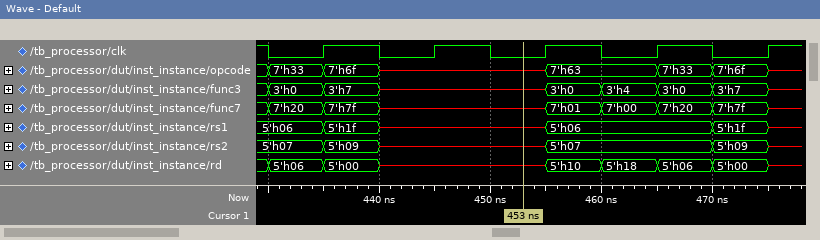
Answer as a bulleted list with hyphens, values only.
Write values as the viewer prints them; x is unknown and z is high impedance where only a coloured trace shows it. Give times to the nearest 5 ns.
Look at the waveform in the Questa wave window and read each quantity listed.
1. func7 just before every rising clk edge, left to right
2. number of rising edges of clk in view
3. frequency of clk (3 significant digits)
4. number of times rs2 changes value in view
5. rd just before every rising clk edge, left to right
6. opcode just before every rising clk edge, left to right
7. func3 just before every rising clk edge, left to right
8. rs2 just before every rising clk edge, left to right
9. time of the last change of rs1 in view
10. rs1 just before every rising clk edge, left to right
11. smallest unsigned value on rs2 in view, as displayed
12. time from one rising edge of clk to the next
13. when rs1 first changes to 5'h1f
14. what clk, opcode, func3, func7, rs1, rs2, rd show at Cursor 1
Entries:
- 7'h20, x, x, 7'h00, 7'h7f
- 5
- 100 MHz
- 5
- 5'h06, x, x, 5'h18, 5'h00
- 7'h33, x, x, 7'h63, 7'h6f
- 3'h0, x, x, 3'h4, 3'h7
- 5'h07, x, x, 5'h07, 5'h09
- 475 ns
- 5'h06, x, x, 5'h06, 5'h1f
- 5'h07
- 10 ns
- 435 ns
- clk=0, opcode=x, func3=x, func7=x, rs1=x, rs2=x, rd=x
